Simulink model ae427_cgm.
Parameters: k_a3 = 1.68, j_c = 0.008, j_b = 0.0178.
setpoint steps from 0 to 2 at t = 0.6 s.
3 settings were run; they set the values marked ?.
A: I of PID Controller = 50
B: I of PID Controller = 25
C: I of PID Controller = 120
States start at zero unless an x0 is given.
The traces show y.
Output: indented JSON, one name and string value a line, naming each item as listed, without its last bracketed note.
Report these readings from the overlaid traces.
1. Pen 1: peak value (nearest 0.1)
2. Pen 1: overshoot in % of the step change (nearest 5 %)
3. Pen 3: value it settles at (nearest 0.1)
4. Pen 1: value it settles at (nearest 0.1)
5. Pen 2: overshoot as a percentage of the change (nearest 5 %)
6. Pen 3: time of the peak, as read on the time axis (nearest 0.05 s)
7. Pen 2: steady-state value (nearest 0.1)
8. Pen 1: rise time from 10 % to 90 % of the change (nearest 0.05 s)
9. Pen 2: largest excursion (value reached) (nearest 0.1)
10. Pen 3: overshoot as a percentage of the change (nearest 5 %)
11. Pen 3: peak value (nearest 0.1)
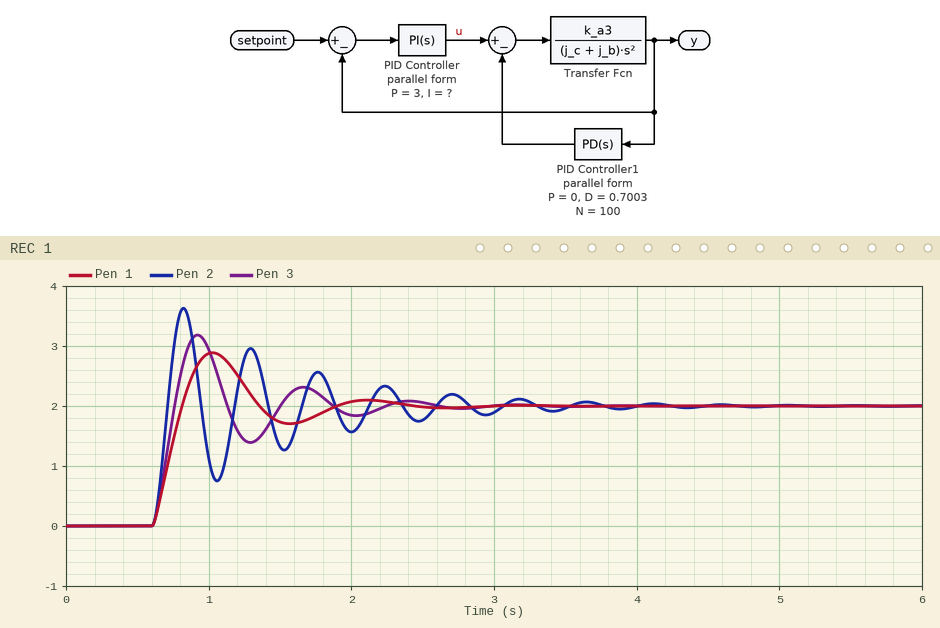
{
  "Pen 1: peak value": "2.9",
  "Pen 1: overshoot in % of the step change": "45 %",
  "Pen 3: value it settles at": "2.0",
  "Pen 1: value it settles at": "2.0",
  "Pen 2: overshoot as a percentage of the change": "80 %",
  "Pen 3: time of the peak, as read on the time axis": "0.90 s",
  "Pen 2: steady-state value": "2.0",
  "Pen 1: rise time from 10 % to 90 % of the change": "0.15 s",
  "Pen 2: largest excursion (value reached)": "3.6",
  "Pen 3: overshoot as a percentage of the change": "60 %",
  "Pen 3: peak value": "3.2"
}
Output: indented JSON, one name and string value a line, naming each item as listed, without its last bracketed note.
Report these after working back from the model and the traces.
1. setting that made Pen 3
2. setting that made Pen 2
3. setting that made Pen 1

{
  "setting that made Pen 3": "A",
  "setting that made Pen 2": "C",
  "setting that made Pen 1": "B"
}
